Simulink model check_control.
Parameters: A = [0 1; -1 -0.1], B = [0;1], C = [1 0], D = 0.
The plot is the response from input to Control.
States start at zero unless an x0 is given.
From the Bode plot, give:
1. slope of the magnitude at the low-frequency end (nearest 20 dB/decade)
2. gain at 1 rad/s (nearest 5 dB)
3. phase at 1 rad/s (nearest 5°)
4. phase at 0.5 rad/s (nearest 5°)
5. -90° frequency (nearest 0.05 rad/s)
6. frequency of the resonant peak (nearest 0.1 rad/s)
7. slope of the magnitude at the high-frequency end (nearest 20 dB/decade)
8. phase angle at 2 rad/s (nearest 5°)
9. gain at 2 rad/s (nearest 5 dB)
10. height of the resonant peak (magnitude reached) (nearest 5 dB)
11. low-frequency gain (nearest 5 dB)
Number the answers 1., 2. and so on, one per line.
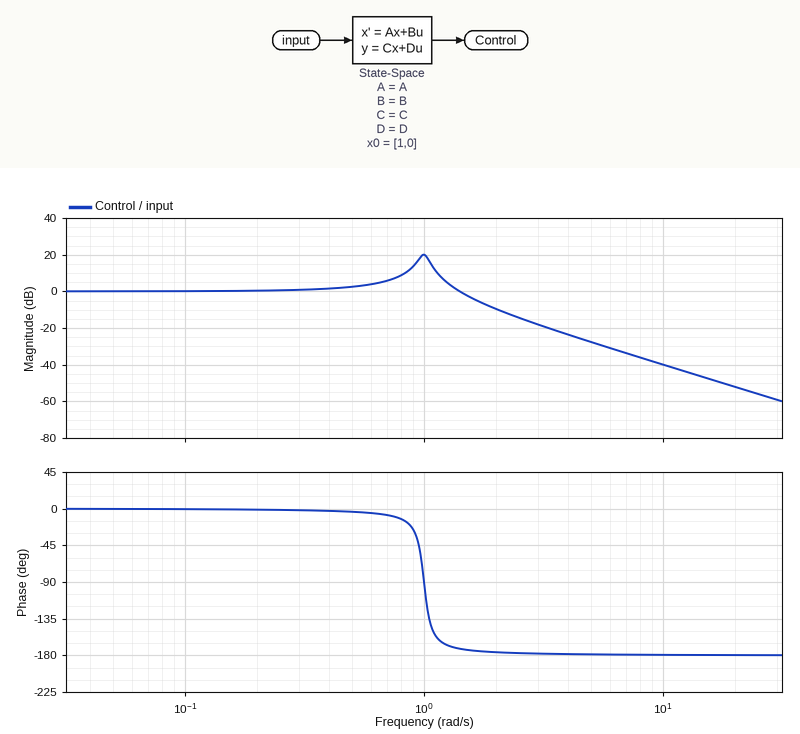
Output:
1. 0 dB/decade
2. 20 dB
3. -90°
4. -5°
5. 1.00 rad/s
6. 1.0 rad/s
7. -40 dB/decade
8. -175°
9. -10 dB
10. 20 dB
11. 0 dB
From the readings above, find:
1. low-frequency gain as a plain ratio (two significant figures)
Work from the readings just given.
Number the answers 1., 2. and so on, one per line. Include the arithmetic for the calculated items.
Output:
1. 10^(0 / 20) = 1.0
